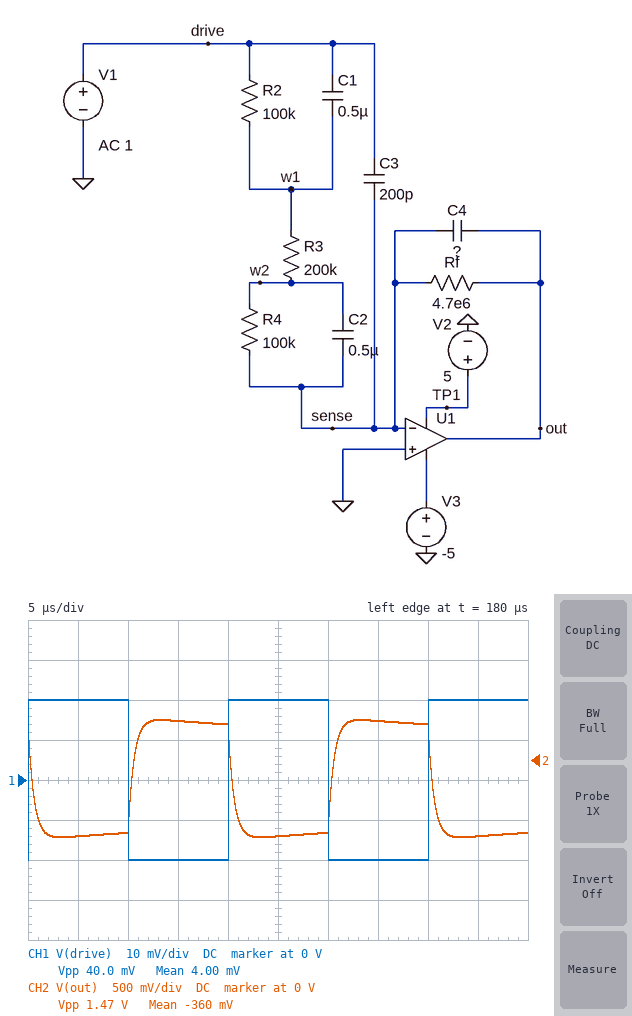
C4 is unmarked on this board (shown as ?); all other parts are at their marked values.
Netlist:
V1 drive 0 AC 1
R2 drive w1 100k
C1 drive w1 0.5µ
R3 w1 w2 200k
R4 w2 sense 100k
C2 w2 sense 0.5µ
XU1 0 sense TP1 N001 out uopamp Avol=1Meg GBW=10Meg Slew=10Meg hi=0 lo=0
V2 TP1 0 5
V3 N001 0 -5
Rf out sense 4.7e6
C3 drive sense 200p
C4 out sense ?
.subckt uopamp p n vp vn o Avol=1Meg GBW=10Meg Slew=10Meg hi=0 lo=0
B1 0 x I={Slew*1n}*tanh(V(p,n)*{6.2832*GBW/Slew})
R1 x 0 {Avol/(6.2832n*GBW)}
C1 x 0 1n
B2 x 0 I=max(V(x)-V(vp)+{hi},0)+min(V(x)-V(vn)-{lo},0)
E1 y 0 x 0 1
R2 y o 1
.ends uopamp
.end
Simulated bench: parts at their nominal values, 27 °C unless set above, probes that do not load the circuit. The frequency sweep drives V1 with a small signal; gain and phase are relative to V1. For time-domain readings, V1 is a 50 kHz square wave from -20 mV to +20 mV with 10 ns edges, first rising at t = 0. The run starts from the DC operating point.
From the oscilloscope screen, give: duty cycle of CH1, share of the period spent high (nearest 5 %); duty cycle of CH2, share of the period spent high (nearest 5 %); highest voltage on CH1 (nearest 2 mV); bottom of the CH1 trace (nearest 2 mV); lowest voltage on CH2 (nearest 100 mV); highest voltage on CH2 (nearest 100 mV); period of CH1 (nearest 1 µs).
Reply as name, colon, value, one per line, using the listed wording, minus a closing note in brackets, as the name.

duty cycle of CH1, share of the period spent high: 50 %
duty cycle of CH2, share of the period spent high: 50 %
highest voltage on CH1: 20 mV
bottom of the CH1 trace: -20 mV
lowest voltage on CH2: -1.0 V
highest voltage on CH2: 500 mV
period of CH1: 20 µs
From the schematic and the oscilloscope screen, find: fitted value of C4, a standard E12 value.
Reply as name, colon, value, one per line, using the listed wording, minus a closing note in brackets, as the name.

fitted value of C4, a standard E12 value: 5.6 pF
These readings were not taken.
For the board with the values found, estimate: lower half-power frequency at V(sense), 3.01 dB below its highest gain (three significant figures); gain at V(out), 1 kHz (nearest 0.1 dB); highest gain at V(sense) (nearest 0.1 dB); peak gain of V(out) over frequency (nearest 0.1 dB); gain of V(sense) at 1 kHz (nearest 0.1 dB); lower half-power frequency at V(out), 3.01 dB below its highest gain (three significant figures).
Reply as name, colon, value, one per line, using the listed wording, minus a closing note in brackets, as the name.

lower half-power frequency at V(sense), 3.01 dB below its highest gain: 270 kHz
gain at V(out), 1 kHz: 27.6 dB
highest gain at V(sense): -0.2 dB
peak gain of V(out) over frequency: 31.0 dB
gain of V(sense) at 1 kHz: -52.4 dB
lower half-power frequency at V(out), 3.01 dB below its highest gain: 2.01 kHz
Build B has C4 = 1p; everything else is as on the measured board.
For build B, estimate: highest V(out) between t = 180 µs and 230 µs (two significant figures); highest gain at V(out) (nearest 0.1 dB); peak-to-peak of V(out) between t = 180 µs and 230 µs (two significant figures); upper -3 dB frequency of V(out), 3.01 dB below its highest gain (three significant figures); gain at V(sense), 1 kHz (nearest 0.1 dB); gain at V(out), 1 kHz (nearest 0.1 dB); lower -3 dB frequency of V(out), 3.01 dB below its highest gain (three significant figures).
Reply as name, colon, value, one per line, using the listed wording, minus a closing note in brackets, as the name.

highest V(out) between t = 180 µs and 230 µs: 3.9 V
highest gain at V(out): 45.4 dB
peak-to-peak of V(out) between t = 180 µs and 230 µs: 8.2 V
upper -3 dB frequency of V(out), 3.01 dB below its highest gain: 75.8 kHz
gain at V(sense), 1 kHz: -52.3 dB
gain at V(out), 1 kHz: 27.7 dB
lower -3 dB frequency of V(out), 3.01 dB below its highest gain: 21.9 kHz
